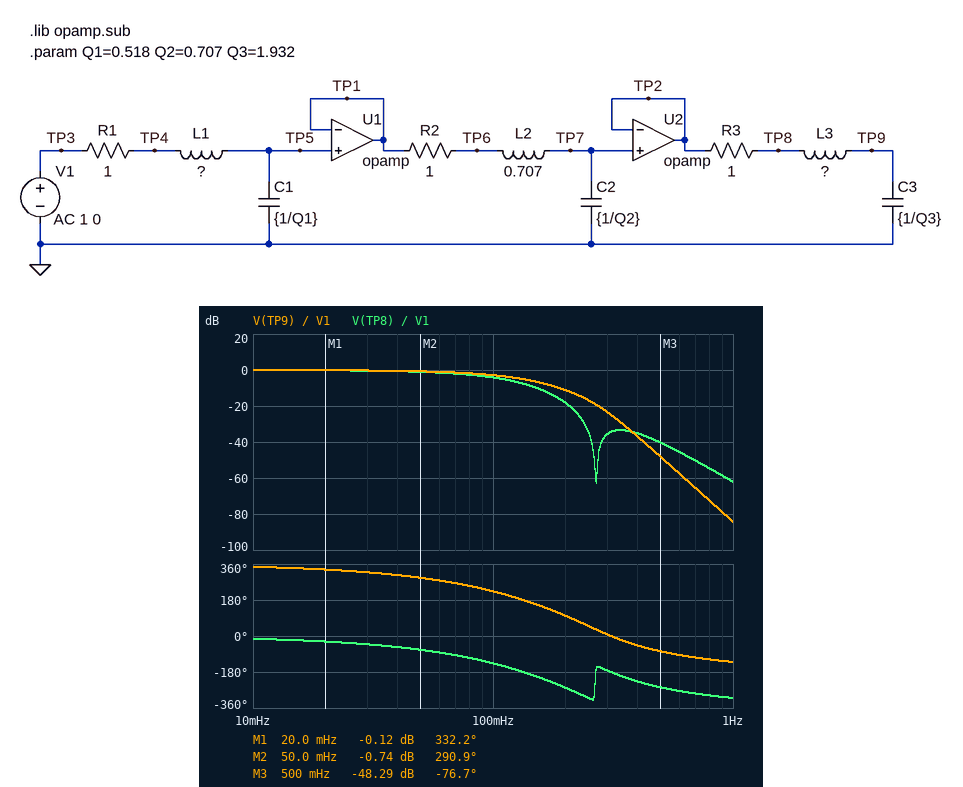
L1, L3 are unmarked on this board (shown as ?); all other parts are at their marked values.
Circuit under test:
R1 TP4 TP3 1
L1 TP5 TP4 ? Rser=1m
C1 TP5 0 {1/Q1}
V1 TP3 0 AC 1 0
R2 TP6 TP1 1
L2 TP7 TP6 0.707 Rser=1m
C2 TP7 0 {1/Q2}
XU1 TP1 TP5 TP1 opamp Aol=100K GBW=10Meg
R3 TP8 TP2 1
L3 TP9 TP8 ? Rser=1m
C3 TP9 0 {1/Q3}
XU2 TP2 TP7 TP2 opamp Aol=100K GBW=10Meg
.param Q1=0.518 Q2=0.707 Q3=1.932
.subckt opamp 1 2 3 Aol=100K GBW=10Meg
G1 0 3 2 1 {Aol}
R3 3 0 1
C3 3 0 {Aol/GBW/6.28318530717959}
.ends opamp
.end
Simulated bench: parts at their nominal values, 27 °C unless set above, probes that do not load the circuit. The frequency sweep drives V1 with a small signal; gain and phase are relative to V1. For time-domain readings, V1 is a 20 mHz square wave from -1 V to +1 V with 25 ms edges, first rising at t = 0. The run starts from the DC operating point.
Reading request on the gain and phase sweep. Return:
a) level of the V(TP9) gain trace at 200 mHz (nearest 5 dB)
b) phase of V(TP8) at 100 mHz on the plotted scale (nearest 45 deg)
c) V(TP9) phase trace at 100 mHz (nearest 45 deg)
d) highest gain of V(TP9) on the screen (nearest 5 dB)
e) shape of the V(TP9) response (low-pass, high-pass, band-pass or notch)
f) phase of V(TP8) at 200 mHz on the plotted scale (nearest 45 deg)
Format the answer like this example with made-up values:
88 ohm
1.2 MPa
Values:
-10 dB
-135 deg
225 deg
0 dB
low-pass
-270 deg
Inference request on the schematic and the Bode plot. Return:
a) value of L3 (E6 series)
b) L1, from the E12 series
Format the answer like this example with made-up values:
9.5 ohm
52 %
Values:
680 mH
390 mH
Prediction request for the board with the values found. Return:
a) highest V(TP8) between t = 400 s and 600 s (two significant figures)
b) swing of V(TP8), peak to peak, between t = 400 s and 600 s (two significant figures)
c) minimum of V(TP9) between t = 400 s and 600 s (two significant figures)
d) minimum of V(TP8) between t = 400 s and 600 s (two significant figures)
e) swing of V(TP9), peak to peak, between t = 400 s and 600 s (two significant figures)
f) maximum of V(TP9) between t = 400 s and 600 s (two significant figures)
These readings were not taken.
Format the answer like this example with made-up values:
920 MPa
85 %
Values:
1.0 V
2.0 V
-1.0 V
-1.0 V
2.0 V
1.0 V
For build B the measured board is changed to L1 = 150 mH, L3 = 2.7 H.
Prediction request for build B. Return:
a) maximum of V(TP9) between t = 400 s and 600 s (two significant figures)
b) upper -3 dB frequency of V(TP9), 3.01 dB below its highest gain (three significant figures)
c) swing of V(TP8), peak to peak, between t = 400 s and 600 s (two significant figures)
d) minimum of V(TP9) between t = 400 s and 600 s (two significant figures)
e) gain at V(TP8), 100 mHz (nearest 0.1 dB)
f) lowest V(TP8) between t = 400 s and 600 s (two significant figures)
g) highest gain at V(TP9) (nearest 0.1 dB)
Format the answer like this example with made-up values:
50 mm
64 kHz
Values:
1.3 V
144 mHz
2.2 V
-1.3 V
-6.0 dB
-1.1 V
1.4 dB
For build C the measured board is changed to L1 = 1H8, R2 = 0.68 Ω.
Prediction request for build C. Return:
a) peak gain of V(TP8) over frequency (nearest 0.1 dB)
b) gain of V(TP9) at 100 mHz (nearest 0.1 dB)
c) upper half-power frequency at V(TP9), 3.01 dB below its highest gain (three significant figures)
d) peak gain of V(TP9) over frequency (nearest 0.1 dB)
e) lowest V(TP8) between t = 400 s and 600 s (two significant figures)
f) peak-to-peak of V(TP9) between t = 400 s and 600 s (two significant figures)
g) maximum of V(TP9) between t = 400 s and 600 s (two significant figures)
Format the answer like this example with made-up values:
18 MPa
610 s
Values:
1.5 dB
0 dB
109 mHz
2.0 dB
-1.4 V
2.9 V
1.5 V
